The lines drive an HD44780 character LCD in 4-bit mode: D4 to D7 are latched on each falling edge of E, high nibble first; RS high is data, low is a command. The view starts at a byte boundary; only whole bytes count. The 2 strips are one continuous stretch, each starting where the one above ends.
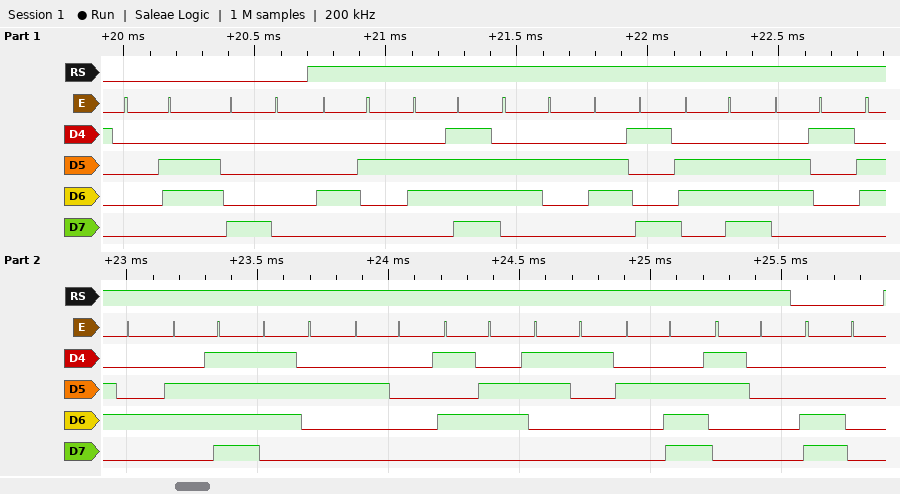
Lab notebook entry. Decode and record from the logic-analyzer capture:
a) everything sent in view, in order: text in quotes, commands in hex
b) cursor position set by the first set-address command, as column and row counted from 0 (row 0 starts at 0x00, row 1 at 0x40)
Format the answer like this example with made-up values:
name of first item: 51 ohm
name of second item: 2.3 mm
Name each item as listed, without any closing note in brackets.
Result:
everything sent in view, in order: text in quotes, commands in hex: 0x06 0x80 "Bobinador V1.0" 0xC0
cursor position set by the first set-address command, as column and row counted from 0: column 0, row 0
